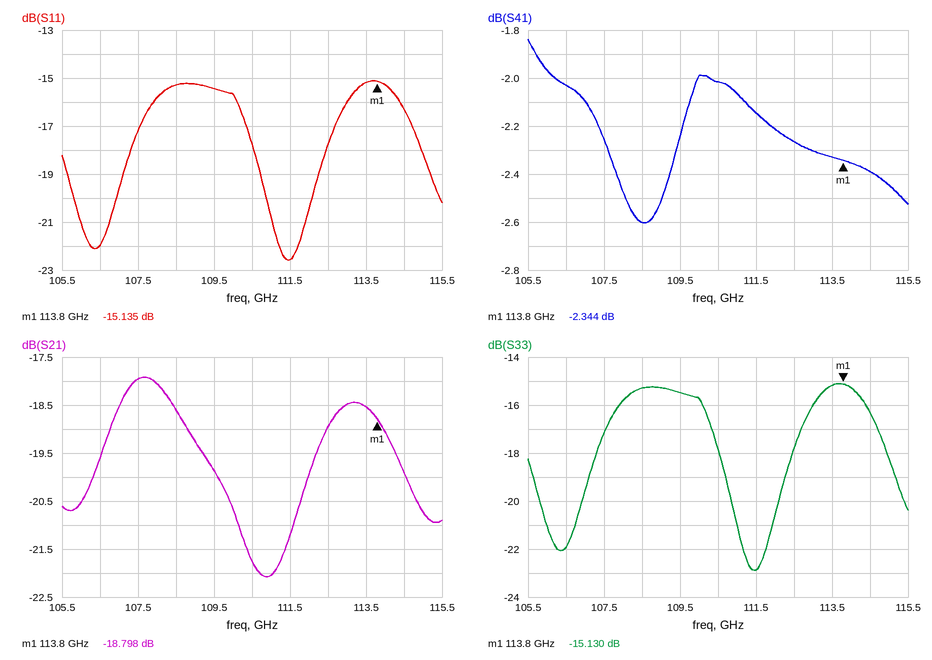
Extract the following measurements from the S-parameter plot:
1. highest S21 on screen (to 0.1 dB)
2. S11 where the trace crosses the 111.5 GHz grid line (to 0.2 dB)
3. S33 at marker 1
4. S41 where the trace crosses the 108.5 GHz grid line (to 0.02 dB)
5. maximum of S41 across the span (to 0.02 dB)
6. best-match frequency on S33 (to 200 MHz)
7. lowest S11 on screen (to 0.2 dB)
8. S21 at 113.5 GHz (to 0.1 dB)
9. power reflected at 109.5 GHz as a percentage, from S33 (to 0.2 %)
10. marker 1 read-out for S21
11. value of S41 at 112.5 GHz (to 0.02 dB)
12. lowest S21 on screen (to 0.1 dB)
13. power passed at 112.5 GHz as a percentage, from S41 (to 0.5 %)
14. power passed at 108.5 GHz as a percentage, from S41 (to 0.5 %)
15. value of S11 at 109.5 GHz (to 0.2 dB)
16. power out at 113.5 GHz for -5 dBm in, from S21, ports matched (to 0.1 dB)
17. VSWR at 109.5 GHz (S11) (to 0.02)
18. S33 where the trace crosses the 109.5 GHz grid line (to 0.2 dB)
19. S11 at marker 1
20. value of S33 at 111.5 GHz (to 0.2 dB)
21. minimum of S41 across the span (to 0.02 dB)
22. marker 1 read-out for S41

-17.9 dB
-22.6 dB
-15.130 dB
-2.60 dB
-1.84 dB
111.4 GHz
-22.6 dB
-18.5 dB
2.8 %
-18.798 dB
-2.26 dB
-22.1 dB
59.5 %
55.0 %
-15.4 dB
-23.5 dBm
1.40
-15.4 dB
-15.135 dB
-22.8 dB
-2.60 dB
-2.344 dB
